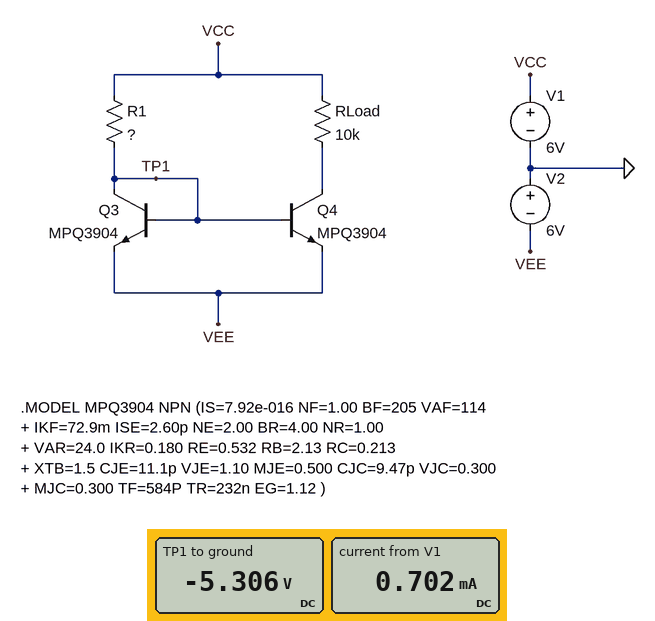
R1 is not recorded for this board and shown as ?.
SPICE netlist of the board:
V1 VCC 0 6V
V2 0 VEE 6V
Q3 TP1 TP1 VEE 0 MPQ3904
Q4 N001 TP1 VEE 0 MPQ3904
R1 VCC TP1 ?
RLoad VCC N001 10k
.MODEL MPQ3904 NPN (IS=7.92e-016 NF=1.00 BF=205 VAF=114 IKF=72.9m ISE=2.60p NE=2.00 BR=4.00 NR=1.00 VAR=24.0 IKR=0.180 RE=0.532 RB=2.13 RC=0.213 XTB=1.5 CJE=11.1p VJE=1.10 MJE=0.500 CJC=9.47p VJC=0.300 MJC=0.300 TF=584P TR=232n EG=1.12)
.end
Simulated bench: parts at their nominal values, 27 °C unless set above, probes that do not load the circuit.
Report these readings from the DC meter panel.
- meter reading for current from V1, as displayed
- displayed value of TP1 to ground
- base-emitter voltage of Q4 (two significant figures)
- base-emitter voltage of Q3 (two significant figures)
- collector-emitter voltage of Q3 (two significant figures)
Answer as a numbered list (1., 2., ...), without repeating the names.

1. 0.702 mA
2. -5.306 V
3. 690 mV
4. 690 mV
5. 690 mV
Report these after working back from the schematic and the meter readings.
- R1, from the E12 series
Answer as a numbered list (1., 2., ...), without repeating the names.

1. 33 kΩ
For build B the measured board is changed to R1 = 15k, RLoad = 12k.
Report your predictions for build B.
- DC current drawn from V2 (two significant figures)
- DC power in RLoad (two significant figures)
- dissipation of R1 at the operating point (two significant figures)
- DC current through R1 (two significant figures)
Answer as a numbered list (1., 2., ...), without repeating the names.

1. 1.5 mA
2. 6.8 mW
3. 8.5 mW
4. 750 µA
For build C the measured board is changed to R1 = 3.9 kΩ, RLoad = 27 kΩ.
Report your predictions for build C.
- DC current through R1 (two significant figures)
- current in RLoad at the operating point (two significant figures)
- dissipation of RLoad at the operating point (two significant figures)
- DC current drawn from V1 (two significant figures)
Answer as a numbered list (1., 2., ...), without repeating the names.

1. 2.9 mA
2. 440 µA
3. 5.3 mW
4. 3.3 mA
